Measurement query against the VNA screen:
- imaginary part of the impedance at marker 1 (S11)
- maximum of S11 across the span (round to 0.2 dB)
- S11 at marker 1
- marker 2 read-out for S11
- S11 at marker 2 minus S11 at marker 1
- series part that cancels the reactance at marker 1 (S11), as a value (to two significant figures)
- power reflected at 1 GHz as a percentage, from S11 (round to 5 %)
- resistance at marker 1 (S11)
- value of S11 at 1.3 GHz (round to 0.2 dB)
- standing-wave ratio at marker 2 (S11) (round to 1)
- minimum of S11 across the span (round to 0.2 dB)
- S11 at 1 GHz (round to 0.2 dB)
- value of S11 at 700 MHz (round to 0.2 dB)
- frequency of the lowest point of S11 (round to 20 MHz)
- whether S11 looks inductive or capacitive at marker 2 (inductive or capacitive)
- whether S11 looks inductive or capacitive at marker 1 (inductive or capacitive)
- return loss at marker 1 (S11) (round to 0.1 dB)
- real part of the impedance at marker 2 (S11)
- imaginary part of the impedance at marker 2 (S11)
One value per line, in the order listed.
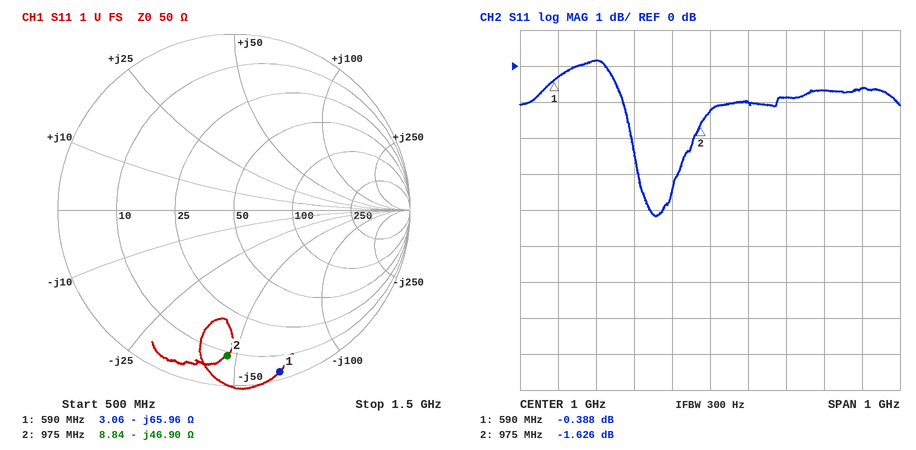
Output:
-65.96 Ω
0.2 dB
-0.388 dB
-1.626 dB
-1.238 dB
18 nH
75 %
3.06 Ω
-0.6 dB
11
-4.2 dB
-1.2 dB
0.2 dB
860 MHz
capacitive
capacitive
0.4 dB
8.84 Ω
-46.90 Ω
